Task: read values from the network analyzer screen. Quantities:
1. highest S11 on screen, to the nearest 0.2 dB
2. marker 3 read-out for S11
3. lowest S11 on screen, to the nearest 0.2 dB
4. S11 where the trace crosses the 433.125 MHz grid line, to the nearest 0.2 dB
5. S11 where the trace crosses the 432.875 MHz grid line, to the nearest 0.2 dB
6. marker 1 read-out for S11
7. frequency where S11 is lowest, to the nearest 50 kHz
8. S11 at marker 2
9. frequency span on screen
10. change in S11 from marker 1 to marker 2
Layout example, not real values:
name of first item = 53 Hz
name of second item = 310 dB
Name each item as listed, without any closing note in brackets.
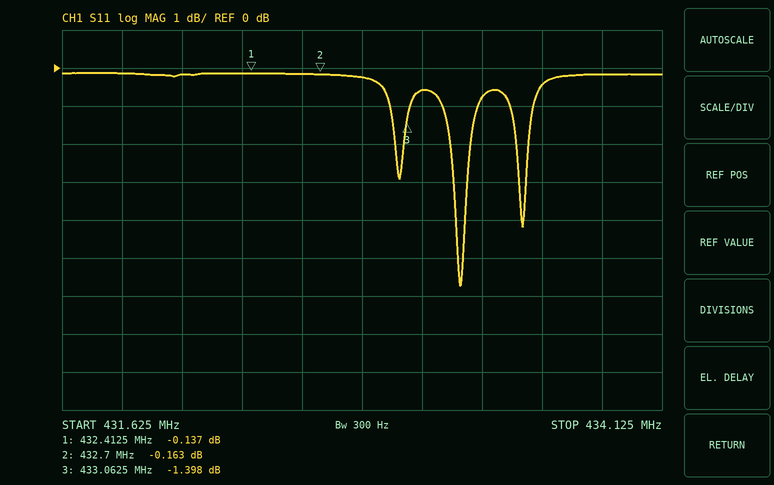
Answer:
highest S11 on screen, to the nearest 0.2 dB = -0.2 dB
marker 3 read-out for S11 = -1.398 dB
lowest S11 on screen, to the nearest 0.2 dB = -5.8 dB
S11 where the trace crosses the 433.125 MHz grid line, to the nearest 0.2 dB = -0.6 dB
S11 where the trace crosses the 432.875 MHz grid line, to the nearest 0.2 dB = -0.2 dB
marker 1 read-out for S11 = -0.137 dB
frequency where S11 is lowest, to the nearest 50 kHz = 433.30 MHz
S11 at marker 2 = -0.163 dB
frequency span on screen = 2.5 MHz
change in S11 from marker 1 to marker 2 = -0.026 dB
